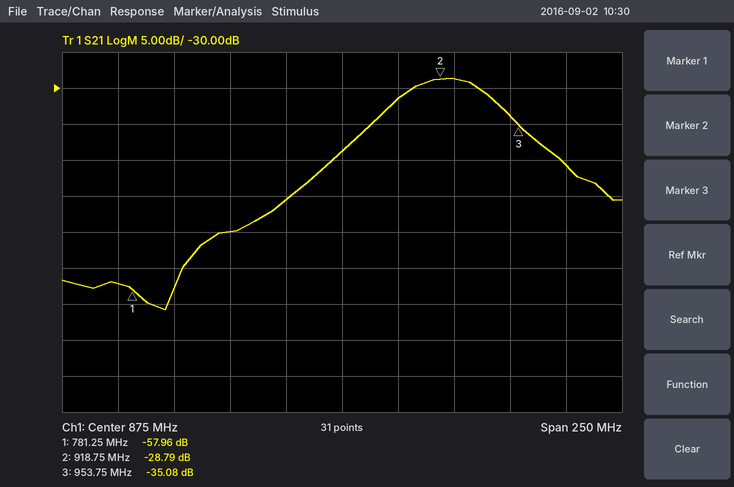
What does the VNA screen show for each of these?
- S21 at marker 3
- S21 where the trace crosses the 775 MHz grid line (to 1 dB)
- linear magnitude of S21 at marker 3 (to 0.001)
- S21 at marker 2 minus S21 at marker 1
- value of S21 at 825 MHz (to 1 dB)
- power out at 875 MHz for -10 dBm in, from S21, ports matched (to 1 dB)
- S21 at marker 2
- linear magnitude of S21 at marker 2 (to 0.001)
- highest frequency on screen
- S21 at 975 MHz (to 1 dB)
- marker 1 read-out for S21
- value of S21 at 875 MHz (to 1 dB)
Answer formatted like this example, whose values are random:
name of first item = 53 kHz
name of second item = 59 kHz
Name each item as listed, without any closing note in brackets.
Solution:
S21 at marker 3 = -35.08 dB
S21 where the trace crosses the 775 MHz grid line = -57 dB
linear magnitude of S21 at marker 3 = 0.018
S21 at marker 2 minus S21 at marker 1 = 29.17 dB
value of S21 at 825 MHz = -50 dB
power out at 875 MHz for -10 dBm in, from S21, ports matched = -49 dBm
S21 at marker 2 = -28.79 dB
linear magnitude of S21 at marker 2 = 0.036
highest frequency on screen = 1 GHz
S21 at 975 MHz = -41 dB
marker 1 read-out for S21 = -57.96 dB
value of S21 at 875 MHz = -39 dB
